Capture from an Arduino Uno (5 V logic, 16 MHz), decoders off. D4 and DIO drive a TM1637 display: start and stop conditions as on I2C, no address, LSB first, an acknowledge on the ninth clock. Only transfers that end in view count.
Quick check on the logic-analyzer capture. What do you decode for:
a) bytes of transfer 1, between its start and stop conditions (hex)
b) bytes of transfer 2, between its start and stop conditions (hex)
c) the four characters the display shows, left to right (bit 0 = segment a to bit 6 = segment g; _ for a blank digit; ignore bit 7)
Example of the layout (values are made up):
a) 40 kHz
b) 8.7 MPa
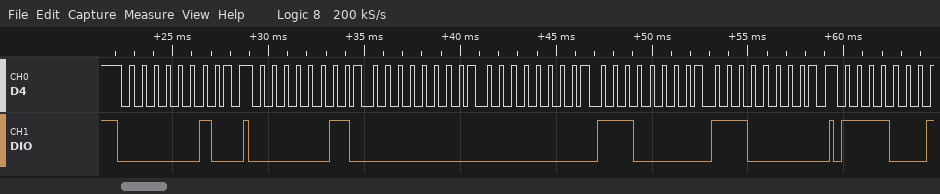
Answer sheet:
a) 40
b) C0 00 00 07 07
c) __77
